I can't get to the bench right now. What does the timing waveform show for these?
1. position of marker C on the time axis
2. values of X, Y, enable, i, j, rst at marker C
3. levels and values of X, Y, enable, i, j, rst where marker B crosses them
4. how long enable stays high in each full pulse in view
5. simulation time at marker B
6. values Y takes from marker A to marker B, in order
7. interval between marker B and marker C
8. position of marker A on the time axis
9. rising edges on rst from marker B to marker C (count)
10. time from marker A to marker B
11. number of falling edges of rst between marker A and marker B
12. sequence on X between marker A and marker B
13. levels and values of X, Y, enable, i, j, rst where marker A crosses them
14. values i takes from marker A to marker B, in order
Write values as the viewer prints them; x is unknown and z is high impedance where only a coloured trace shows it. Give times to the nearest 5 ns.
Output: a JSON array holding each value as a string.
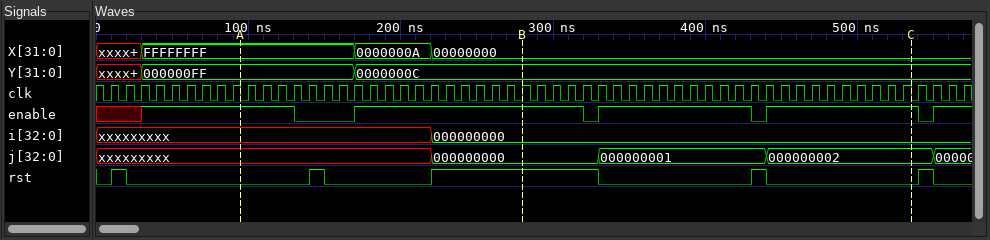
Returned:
["535 ns", "X=00000000, Y=0000000C, enable=1, i=000000000, j=000000002, rst=0", "X=00000000, Y=0000000C, enable=1, i=000000000, j=000000000, rst=1", "150 ns, 100 ns, 100 ns", "280 ns", "000000FF, 0000000C", "255 ns", "95 ns", "1", "185 ns", "1", "FFFFFFFF, 0000000A, 00000000", "X=FFFFFFFF, Y=000000FF, enable=1, i=xxxxxxxxx, j=xxxxxxxxx, rst=0", "xxxxxxxxx, 000000000"]
